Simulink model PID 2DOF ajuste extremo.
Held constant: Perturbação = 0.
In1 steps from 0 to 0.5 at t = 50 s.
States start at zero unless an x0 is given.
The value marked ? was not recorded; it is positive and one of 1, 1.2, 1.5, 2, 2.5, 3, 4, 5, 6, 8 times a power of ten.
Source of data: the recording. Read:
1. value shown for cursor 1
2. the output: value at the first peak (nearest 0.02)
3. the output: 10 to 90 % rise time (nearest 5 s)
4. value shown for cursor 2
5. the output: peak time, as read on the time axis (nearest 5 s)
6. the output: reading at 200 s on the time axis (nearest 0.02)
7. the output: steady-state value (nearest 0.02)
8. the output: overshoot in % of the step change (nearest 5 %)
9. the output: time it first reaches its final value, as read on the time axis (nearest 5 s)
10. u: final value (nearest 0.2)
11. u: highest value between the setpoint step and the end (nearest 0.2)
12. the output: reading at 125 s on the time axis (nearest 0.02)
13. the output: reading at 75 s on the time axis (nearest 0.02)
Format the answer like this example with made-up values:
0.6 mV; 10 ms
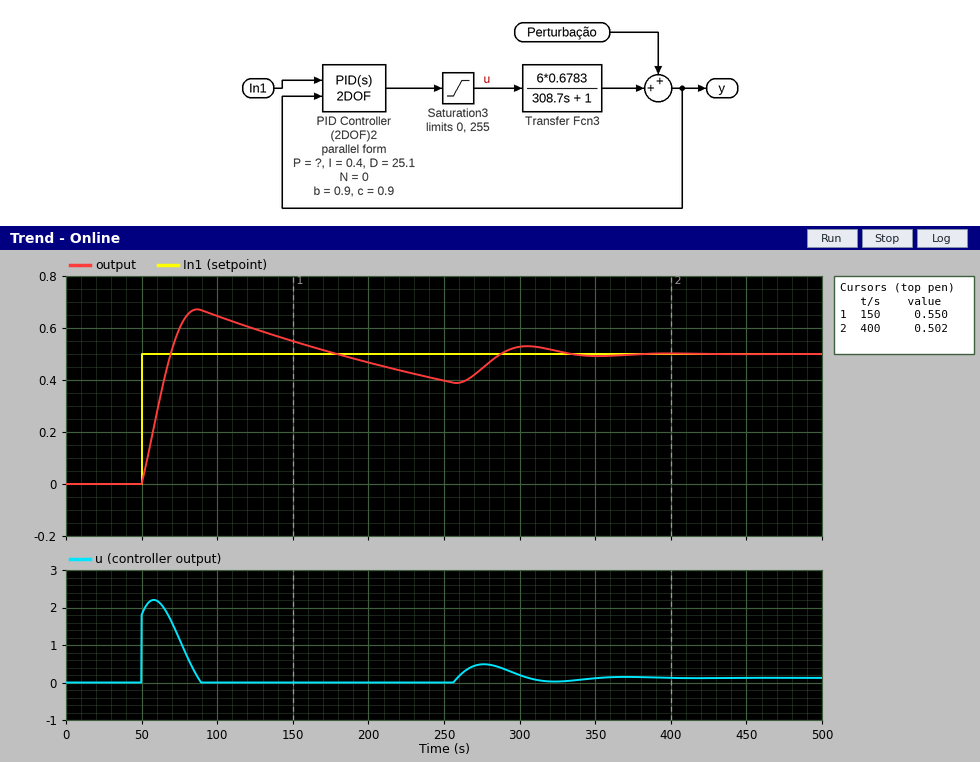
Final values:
0.550; 0.68; 15 s; 0.502; 85 s; 0.46; 0.50; 35 %; 70 s; 0.2; 2.2; 0.60; 0.60
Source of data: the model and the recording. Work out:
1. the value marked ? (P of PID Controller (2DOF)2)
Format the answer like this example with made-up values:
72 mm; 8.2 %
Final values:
4
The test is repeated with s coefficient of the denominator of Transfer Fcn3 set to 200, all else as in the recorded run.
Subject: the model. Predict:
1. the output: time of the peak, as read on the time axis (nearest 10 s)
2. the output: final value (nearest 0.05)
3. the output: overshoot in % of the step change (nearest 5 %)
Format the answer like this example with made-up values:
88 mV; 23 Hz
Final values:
80 s; 0.50; 25 %
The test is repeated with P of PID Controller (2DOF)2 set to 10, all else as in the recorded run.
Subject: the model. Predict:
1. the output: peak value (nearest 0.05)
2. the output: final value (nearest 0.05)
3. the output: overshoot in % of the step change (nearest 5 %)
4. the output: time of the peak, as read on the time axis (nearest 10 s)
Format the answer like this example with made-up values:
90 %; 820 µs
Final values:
0.55; 0.50; 10 %; 80 s
